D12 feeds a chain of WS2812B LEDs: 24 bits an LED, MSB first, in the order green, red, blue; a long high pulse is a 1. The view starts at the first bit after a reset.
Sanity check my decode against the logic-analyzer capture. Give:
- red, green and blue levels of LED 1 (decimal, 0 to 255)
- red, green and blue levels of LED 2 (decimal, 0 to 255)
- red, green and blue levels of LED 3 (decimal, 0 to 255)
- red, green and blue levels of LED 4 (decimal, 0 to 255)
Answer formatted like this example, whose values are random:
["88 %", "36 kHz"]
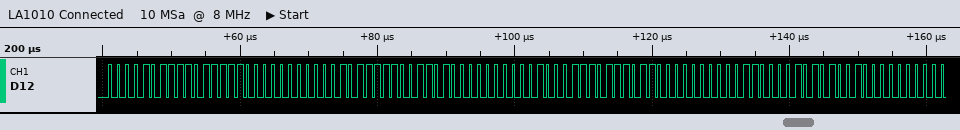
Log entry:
["223, 11, 0", "205, 23, 0", "187, 35, 0", "169, 48, 0"]
